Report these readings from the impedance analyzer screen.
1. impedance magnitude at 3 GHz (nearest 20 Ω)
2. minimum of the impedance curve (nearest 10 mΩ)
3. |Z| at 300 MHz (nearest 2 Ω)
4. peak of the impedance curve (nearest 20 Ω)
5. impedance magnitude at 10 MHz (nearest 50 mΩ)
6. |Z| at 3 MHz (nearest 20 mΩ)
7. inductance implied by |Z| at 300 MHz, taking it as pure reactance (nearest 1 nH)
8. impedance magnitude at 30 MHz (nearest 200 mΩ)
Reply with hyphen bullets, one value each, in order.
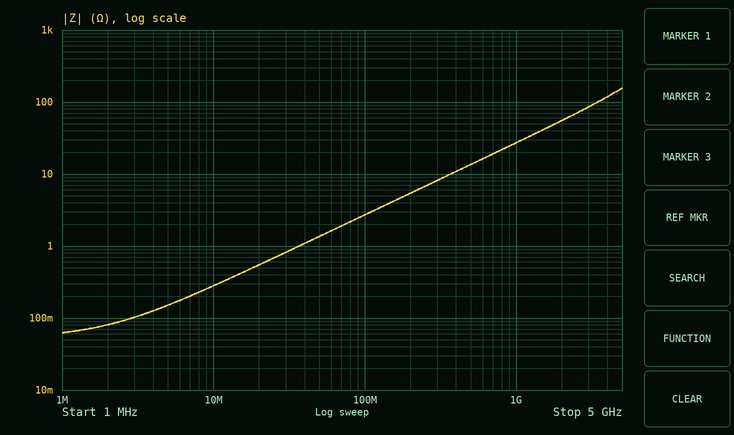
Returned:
- 80 Ω
- 60 mΩ
- 8 Ω
- 160 Ω
- 300 mΩ
- 100 mΩ
- 4 nH
- 800 mΩ
